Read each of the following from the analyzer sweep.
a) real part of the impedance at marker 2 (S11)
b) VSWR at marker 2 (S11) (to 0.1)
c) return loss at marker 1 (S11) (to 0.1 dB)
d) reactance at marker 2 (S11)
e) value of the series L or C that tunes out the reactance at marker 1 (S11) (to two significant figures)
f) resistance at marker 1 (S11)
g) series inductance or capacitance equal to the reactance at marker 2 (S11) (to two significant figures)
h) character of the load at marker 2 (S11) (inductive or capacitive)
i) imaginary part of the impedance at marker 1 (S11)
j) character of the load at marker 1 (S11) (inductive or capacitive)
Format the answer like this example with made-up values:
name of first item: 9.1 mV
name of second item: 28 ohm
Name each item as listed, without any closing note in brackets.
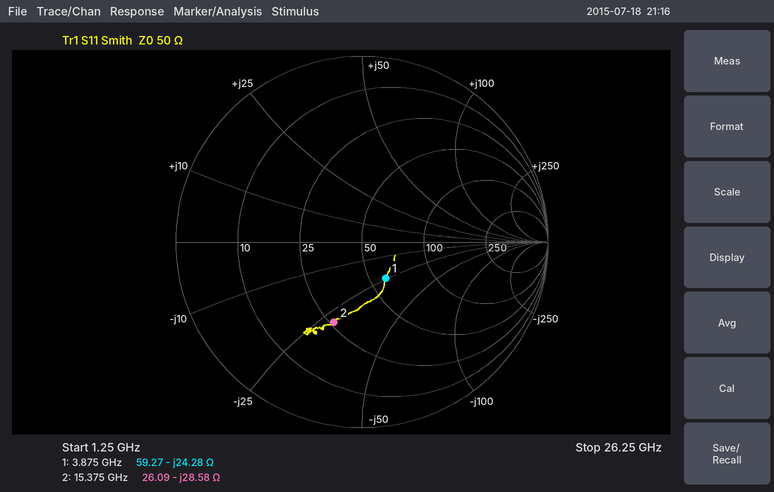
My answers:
real part of the impedance at marker 2: 26.09 Ω
VSWR at marker 2 (S11): 2.7
return loss at marker 1 (S11): 12.7 dB
reactance at marker 2: -28.58 Ω
value of the series L or C that tunes out the reactance at marker 1 (S11): 1.00 nH
resistance at marker 1: 59.27 Ω
series inductance or capacitance equal to the reactance at marker 2 (S11): 360 fF
character of the load at marker 2 (S11): capacitive
imaginary part of the impedance at marker 1: -24.28 Ω
character of the load at marker 1 (S11): capacitive
